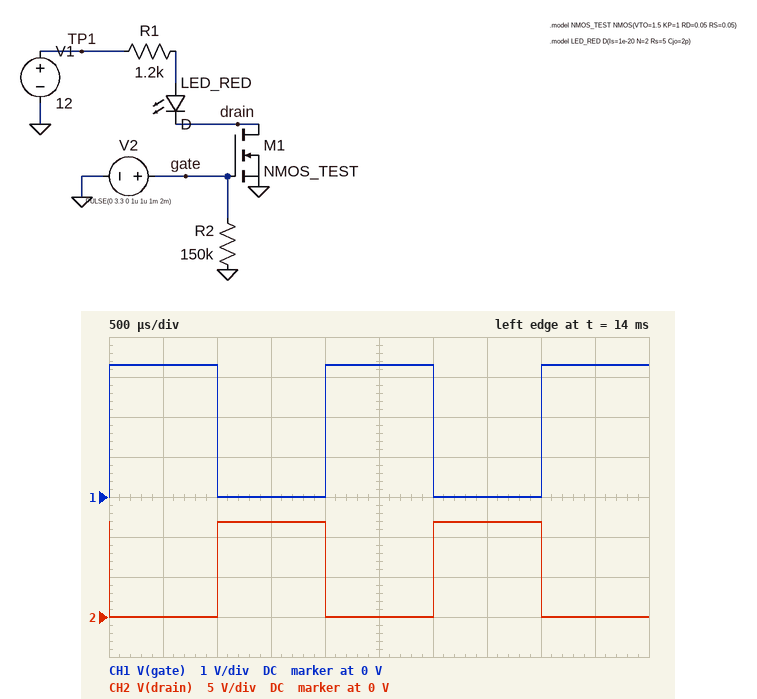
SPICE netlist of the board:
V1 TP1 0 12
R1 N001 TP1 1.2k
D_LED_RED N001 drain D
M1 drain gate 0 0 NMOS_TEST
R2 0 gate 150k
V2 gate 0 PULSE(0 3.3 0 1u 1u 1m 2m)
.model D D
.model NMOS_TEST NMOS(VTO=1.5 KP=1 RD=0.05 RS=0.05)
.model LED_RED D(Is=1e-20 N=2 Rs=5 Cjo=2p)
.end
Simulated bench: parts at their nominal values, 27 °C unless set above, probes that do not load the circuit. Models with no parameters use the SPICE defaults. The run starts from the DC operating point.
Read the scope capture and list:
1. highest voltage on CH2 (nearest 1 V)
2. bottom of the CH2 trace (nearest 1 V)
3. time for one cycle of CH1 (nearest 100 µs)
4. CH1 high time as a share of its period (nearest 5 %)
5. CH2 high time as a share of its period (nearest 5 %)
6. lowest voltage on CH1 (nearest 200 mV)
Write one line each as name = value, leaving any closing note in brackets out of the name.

highest voltage on CH2 = 12 V
bottom of the CH2 trace = 0 V
time for one cycle of CH1 = 2.0 ms
CH1 high time as a share of its period = 50 %
CH2 high time as a share of its period = 50 %
lowest voltage on CH1 = 0 V
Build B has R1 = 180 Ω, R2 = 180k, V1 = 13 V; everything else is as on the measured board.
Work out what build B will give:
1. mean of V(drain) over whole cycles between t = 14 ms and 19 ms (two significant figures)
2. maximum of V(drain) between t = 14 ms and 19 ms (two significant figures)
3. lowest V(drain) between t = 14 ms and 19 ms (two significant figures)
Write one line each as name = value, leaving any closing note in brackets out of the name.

mean of V(drain) over whole cycles between t = 14 ms and 19 ms = 6.4 V
maximum of V(drain) between t = 14 ms and 19 ms = 13 V
lowest V(drain) between t = 14 ms and 19 ms = 45 mV
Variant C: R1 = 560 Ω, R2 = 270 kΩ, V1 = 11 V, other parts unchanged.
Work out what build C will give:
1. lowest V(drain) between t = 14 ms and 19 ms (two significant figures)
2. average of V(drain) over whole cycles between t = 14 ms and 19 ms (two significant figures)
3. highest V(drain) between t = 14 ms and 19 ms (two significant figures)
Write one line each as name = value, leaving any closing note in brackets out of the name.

lowest V(drain) between t = 14 ms and 19 ms = 12 mV
average of V(drain) over whole cycles between t = 14 ms and 19 ms = 5.4 V
highest V(drain) between t = 14 ms and 19 ms = 11 V
